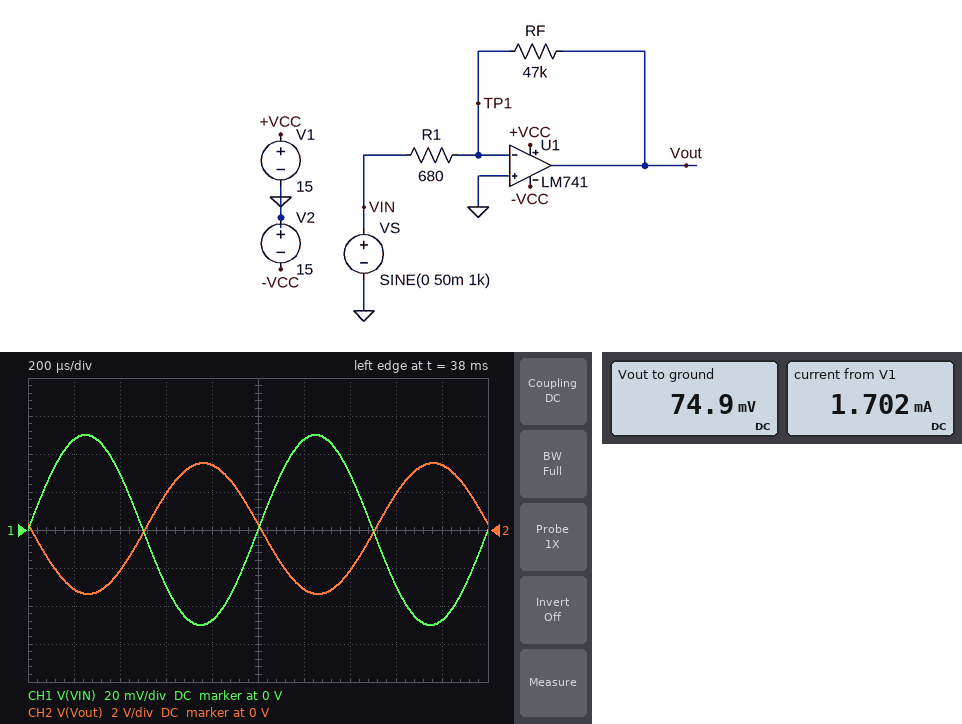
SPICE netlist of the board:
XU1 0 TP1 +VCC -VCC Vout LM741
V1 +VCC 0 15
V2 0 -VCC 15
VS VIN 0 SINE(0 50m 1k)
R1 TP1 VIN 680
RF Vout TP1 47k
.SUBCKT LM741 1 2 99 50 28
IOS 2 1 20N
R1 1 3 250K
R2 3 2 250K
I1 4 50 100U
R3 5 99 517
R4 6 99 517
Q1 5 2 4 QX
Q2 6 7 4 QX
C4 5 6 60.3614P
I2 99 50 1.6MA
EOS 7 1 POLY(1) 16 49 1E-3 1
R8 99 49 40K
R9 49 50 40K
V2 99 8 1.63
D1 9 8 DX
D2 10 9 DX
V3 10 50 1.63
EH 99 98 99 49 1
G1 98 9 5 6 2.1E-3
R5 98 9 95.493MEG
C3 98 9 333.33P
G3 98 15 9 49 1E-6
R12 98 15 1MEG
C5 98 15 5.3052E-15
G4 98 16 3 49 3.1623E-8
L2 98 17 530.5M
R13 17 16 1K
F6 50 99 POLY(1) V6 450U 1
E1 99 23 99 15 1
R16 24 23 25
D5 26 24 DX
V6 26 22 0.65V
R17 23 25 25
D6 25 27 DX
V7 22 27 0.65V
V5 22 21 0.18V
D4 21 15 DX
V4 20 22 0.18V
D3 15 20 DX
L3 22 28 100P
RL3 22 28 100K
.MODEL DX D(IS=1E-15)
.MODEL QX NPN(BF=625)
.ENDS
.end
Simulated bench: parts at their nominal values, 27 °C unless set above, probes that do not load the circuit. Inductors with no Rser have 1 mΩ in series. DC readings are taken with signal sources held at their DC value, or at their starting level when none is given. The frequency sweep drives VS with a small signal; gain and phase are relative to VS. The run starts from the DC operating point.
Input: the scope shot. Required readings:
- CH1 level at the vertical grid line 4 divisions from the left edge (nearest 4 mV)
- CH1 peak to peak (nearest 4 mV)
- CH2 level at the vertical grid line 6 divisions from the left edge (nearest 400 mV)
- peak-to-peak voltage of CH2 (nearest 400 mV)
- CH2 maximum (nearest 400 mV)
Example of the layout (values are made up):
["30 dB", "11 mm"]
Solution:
["-48 mV", "100 mV", "-3.2 V", "6.8 V", "3.6 V"]
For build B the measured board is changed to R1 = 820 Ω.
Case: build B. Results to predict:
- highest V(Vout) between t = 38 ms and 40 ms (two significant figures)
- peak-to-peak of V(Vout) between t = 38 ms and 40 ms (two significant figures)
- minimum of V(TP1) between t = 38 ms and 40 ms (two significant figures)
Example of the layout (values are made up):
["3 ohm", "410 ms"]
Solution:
["2.9 V", "5.7 V", "-1.9 mV"]
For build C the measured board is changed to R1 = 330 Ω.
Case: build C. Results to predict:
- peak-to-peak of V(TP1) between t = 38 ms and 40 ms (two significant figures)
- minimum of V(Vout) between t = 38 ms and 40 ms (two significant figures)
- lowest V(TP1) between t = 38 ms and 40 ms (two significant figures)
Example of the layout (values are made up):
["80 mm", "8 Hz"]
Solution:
["14 mV", "-6.9 V", "-6.1 mV"]
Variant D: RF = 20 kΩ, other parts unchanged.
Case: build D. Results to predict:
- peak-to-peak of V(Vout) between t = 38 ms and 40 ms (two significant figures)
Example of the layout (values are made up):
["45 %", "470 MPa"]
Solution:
["2.9 V"]
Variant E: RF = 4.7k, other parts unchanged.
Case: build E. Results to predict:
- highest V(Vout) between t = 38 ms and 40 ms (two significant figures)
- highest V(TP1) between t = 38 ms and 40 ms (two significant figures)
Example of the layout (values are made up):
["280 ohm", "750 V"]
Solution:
["350 mV", "1.4 mV"]
